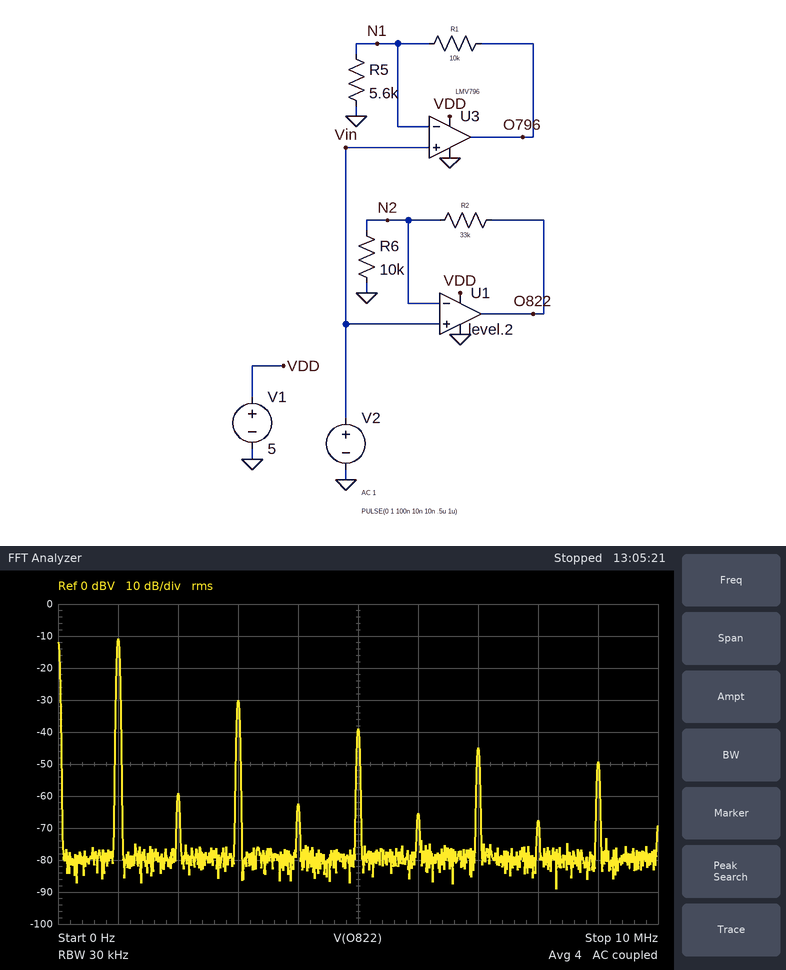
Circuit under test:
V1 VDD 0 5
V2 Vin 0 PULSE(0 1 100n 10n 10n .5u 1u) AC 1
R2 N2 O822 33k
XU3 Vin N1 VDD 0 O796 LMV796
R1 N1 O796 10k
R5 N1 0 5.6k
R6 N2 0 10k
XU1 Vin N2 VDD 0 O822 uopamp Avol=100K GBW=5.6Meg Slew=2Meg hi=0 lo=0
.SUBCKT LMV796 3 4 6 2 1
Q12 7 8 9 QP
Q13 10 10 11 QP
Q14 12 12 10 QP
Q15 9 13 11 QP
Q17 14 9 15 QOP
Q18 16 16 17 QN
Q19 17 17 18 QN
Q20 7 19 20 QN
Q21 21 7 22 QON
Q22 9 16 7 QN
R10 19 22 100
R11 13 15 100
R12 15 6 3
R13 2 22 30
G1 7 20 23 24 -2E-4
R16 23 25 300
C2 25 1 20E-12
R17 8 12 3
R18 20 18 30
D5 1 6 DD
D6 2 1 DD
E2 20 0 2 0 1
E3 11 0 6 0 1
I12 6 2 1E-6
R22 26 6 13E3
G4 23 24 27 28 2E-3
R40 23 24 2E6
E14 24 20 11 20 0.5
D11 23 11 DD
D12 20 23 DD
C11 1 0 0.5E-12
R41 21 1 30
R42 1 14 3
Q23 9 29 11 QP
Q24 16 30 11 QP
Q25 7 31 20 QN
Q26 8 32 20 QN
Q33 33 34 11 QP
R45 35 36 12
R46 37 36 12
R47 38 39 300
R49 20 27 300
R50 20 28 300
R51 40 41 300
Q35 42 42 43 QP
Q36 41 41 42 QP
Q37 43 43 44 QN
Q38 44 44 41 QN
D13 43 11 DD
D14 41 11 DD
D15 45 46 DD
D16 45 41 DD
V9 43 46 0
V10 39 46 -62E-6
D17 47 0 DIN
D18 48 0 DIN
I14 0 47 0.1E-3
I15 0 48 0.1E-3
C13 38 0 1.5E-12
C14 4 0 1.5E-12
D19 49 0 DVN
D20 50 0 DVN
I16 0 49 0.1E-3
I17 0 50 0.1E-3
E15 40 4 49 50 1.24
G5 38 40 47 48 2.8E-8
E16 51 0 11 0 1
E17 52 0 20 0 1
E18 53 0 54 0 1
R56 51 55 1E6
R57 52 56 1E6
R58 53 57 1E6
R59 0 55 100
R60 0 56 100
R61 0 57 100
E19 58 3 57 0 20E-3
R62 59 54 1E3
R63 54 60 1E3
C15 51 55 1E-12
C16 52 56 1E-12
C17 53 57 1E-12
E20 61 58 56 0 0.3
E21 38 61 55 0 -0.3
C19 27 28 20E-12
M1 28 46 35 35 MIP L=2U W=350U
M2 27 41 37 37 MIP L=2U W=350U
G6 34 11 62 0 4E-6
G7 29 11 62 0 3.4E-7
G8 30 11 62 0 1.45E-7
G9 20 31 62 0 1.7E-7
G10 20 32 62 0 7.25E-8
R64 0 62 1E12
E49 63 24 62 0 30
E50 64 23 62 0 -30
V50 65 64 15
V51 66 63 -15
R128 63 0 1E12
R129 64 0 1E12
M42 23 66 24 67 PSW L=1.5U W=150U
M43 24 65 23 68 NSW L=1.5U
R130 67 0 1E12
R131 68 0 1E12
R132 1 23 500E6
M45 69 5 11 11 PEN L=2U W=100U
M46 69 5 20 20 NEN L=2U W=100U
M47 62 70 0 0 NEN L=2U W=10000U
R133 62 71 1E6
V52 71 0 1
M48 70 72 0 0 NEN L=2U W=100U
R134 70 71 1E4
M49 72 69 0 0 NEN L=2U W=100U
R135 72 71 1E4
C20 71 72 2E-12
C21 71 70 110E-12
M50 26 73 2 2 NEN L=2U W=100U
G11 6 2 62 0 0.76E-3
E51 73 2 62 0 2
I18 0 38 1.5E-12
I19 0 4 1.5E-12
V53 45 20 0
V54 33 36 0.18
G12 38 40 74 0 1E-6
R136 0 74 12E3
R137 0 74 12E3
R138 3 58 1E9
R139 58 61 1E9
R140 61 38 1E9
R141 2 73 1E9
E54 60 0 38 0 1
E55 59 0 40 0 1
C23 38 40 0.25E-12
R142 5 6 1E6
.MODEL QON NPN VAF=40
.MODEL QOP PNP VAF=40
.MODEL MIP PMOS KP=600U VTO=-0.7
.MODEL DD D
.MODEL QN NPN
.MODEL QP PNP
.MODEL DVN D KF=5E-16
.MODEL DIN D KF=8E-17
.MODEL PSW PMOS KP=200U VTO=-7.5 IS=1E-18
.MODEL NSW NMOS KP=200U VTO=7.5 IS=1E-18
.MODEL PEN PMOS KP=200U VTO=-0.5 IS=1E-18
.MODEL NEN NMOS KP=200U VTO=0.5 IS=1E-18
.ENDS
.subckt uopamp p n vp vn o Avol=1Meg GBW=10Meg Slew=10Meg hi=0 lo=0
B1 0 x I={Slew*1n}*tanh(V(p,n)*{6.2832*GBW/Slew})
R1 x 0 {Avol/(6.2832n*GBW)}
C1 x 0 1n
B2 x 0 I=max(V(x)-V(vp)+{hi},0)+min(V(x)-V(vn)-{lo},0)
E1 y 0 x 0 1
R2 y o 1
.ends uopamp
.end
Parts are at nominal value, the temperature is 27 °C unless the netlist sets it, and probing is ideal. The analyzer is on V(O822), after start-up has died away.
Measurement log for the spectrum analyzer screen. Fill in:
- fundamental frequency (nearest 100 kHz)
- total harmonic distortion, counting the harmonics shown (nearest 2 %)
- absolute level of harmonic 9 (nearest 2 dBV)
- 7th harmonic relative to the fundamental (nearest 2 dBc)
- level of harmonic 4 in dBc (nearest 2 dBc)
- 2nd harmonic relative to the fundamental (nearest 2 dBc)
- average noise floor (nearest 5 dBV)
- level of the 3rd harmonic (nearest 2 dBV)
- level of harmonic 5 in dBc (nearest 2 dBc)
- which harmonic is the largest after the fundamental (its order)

1.0 MHz
12 %
-50 dBV
-34 dBc
-52 dBc
-48 dBc
-80 dBV
-30 dBV
-28 dBc
3
